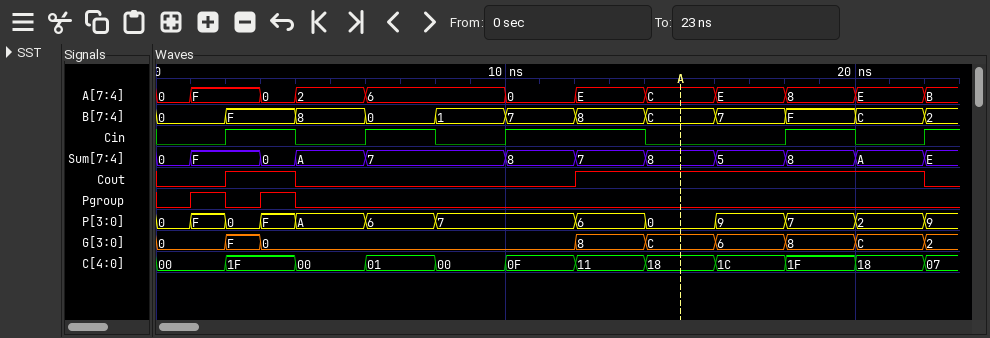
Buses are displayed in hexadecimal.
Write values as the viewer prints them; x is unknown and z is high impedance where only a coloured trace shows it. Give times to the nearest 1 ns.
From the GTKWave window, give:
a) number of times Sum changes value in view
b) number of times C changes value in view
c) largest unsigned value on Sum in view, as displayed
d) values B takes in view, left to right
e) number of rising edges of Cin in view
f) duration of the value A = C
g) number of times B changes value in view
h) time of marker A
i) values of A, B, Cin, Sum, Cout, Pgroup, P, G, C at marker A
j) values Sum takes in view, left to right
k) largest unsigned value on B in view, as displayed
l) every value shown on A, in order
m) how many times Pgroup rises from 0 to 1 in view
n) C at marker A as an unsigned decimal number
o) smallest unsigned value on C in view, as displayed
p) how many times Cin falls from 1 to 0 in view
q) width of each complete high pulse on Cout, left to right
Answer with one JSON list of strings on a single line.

["11", "11", "F", "0, F, 8, 0, 1, 7, 8, C, 7, F, C, 2", "5", "2 ns", "11", "15 ns", "A=C, B=C, Cin=0, Sum=8, Cout=1, Pgroup=0, P=0, G=C, C=18", "0, F, 0, A, 7, 8, 7, 8, 5, 8, A, E", "F", "0, F, 0, 2, 6, 0, E, C, E, 8, E, B", "2", "24", "00", "4", "2 ns, 10 ns"]
